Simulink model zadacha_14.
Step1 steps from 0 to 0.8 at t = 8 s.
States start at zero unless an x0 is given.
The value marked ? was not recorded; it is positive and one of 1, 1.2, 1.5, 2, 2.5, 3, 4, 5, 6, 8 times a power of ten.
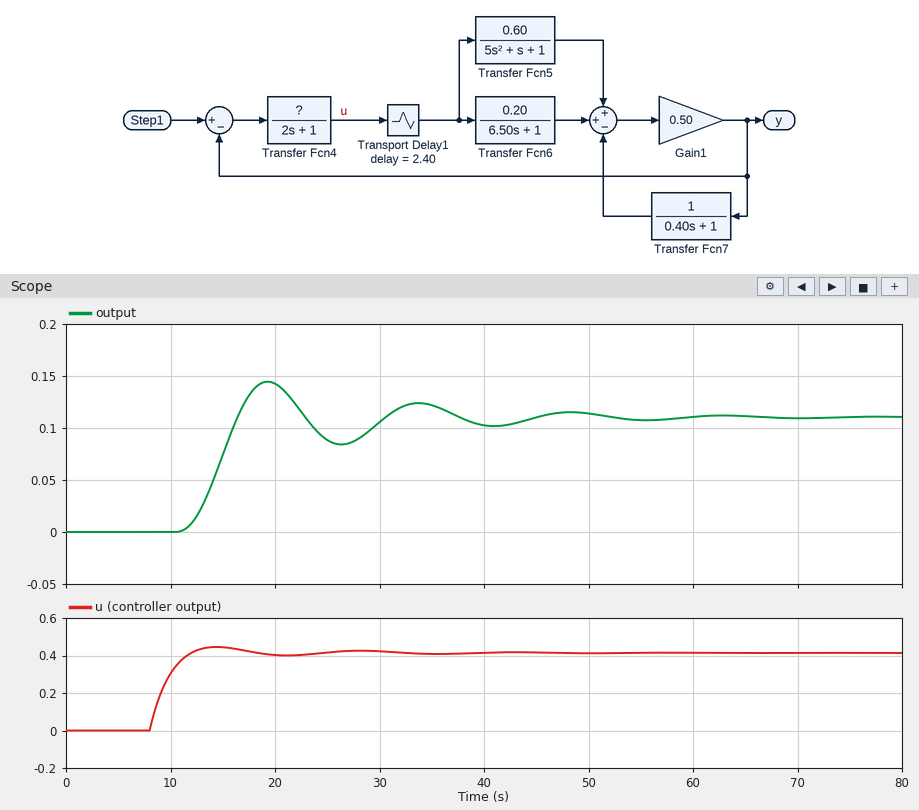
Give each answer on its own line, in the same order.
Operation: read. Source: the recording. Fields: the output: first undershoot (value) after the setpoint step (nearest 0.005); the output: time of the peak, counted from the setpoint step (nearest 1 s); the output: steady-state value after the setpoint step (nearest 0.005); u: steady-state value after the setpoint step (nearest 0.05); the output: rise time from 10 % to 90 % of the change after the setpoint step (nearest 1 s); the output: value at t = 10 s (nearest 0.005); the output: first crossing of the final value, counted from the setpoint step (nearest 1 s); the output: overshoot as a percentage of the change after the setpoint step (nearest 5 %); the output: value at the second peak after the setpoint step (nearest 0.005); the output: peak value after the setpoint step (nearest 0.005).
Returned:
0.085
11 s
0.110
0.40
4 s
0.000
8 s
30 %
0.125
0.145
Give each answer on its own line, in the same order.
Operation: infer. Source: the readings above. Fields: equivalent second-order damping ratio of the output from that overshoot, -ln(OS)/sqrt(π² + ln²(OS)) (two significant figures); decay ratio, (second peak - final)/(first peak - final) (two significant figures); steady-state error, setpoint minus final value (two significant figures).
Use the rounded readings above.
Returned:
0.36
0.43
0.69
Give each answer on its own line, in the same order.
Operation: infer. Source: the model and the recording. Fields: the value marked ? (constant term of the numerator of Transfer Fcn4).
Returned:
0.6
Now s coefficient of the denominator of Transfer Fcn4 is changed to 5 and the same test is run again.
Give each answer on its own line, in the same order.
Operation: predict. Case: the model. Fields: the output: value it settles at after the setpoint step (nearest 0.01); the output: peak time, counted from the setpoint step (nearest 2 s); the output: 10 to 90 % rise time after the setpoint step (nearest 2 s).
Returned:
0.11
14 s
6 s
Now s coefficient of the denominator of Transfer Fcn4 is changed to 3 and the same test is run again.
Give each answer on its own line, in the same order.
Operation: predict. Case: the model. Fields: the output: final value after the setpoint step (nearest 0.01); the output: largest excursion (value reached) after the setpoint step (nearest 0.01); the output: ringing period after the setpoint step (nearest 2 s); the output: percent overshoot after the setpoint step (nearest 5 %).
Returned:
0.11
0.13
14 s
20 %
